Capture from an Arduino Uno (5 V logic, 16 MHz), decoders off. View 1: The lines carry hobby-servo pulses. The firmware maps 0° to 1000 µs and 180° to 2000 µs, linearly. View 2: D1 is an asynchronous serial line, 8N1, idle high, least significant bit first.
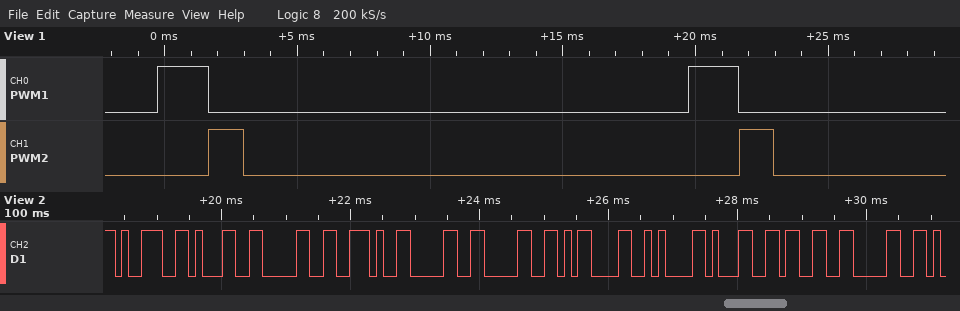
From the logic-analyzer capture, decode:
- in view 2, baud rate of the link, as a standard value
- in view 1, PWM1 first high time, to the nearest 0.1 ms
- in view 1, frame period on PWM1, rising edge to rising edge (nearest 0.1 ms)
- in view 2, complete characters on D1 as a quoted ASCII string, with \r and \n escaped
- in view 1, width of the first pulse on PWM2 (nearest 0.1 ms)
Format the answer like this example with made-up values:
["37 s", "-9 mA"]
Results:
["9600 baud", "1.9 ms", "20.0 ms", "\"910.00\\r\\n130\"", "1.3 ms"]
